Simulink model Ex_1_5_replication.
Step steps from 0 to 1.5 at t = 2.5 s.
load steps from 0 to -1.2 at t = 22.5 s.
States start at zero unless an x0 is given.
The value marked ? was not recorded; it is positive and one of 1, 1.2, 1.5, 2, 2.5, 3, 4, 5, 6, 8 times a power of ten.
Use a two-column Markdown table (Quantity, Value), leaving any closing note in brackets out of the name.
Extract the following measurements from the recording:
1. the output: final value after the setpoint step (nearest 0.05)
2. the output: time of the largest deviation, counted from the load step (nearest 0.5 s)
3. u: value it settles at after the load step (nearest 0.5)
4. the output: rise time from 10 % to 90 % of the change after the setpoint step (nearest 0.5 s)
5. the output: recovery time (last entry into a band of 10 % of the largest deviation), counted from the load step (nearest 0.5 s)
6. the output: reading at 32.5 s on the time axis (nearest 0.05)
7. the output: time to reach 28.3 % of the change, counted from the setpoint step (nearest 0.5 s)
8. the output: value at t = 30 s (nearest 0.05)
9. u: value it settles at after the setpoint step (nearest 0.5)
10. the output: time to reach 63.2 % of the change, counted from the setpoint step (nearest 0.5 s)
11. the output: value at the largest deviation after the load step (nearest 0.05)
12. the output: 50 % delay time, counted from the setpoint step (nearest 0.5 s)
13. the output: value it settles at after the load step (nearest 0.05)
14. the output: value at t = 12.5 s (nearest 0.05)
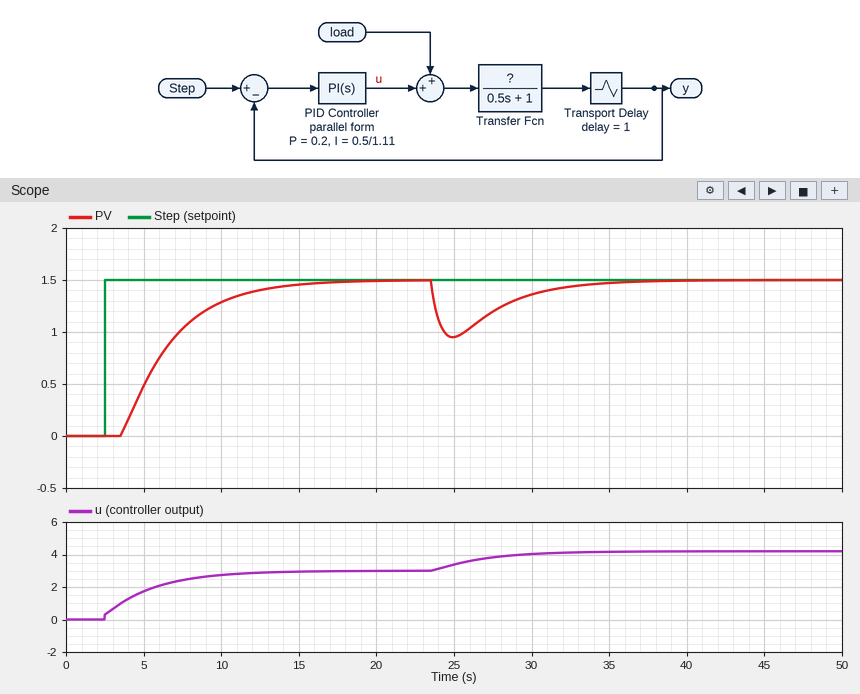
| Quantity | Value |
|---|---|
| the output: final value after the setpoint step | 1.50 |
| the output: time of the largest deviation, counted from the load step | 2.5 s |
| u: value it settles at after the load step | 4.0 |
| the output: rise time from 10 % to 90 % of the change after the setpoint step | 7.0 s |
| the output: recovery time (last entry into a band of 10 % of the largest deviation), counted from the load step | 10.5 s |
| the output: reading at 32.5 s on the time axis | 1.45 |
| the output: time to reach 28.3 % of the change, counted from the setpoint step | 2.5 s |
| the output: value at t = 30 s | 1.35 |
| u: value it settles at after the setpoint step | 3.0 |
| the output: time to reach 63.2 % of the change, counted from the setpoint step | 4.5 s |
| the output: value at the largest deviation after the load step | 0.95 |
| the output: 50 % delay time, counted from the setpoint step | 3.5 s |
| the output: value it settles at after the load step | 1.50 |
| the output: value at t = 12.5 s | 1.40 |
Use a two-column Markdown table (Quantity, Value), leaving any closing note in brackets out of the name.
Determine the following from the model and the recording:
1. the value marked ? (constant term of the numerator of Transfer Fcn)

| Quantity | Value |
|---|---|
| the value marked ? | 0.5 |
